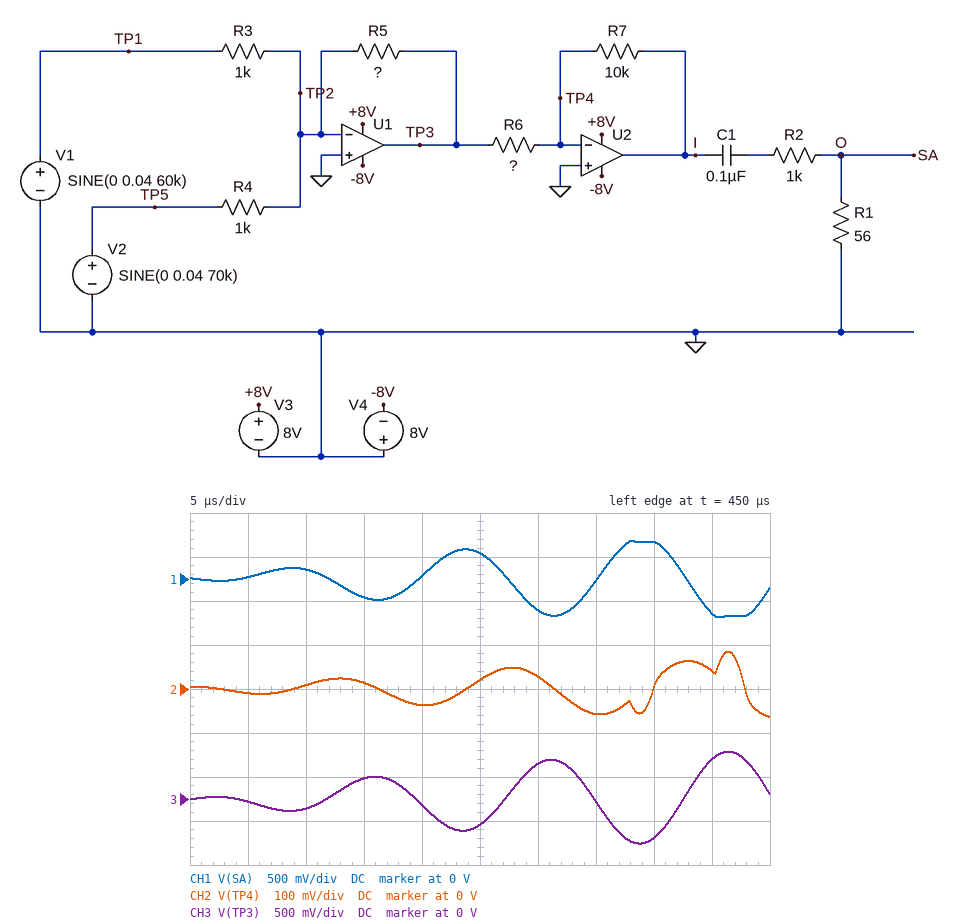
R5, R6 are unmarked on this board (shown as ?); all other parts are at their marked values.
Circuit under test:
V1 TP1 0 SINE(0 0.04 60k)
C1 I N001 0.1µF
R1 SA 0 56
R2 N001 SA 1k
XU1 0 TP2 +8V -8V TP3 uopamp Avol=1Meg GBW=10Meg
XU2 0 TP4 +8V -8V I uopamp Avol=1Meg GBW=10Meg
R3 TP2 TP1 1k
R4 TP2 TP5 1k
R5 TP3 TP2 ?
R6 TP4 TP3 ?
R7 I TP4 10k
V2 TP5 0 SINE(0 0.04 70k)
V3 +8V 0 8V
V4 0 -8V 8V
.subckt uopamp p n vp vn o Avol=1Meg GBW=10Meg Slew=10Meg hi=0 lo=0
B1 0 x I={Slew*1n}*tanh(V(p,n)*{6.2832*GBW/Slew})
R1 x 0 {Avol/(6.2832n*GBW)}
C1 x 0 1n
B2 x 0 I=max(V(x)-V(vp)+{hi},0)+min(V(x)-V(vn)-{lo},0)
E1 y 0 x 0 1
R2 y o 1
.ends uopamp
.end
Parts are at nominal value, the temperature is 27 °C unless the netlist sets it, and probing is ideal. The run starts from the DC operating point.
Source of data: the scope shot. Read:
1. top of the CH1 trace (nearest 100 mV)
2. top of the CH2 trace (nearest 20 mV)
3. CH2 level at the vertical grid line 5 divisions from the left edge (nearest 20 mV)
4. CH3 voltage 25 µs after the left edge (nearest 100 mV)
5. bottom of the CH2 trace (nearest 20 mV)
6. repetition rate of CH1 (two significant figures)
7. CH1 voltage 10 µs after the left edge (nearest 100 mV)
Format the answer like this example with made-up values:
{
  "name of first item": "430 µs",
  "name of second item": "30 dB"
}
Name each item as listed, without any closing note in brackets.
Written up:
{
  "top of the CH1 trace": "400 mV",
  "top of the CH2 trace": "80 mV",
  "CH2 level at the vertical grid line 5 divisions from the left edge": "20 mV",
  "CH3 voltage 25 µs after the left edge": "-300 mV",
  "bottom of the CH2 trace": "-60 mV",
  "repetition rate of CH1": "65 kHz",
  "CH1 voltage 10 µs after the left edge": "100 mV"
}
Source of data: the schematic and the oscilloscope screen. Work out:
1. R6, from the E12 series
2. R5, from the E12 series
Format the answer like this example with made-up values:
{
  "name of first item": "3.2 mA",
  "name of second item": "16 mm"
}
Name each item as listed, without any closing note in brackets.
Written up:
{
  "R6, from the E12 series": "560 Ω",
  "R5, from the E12 series": "6.8 kΩ"
}
